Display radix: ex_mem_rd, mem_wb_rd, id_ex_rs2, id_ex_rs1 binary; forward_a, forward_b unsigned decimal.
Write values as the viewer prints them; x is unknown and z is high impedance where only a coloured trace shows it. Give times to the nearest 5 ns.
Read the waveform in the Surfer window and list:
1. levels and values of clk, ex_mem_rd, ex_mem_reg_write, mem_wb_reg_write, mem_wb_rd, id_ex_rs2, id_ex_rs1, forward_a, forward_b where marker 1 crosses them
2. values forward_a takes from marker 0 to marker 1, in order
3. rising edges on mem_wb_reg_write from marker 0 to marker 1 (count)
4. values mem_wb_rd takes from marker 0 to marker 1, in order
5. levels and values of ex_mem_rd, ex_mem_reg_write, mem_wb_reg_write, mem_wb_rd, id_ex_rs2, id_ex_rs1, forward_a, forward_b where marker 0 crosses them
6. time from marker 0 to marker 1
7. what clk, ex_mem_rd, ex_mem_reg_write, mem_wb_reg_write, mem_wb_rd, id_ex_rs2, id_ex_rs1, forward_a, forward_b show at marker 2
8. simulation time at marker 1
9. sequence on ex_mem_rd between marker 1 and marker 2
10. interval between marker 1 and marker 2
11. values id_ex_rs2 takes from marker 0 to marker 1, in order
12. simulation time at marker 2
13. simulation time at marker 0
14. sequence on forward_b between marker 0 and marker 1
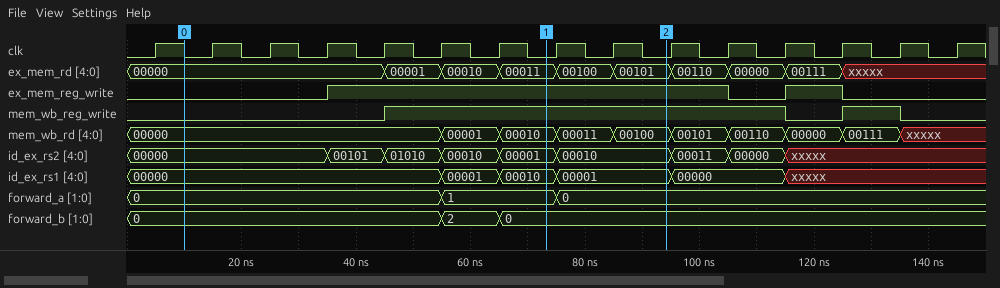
clk=0, ex_mem_rd=00011, ex_mem_reg_write=1, mem_wb_reg_write=1, mem_wb_rd=00010, id_ex_rs2=00001, id_ex_rs1=00010, forward_a=1, forward_b=0
0, 1
1
00000, 00001, 00010
ex_mem_rd=00000, ex_mem_reg_write=0, mem_wb_reg_write=0, mem_wb_rd=00000, id_ex_rs2=00000, id_ex_rs1=00000, forward_a=0, forward_b=0
65 ns
clk=0, ex_mem_rd=00101, ex_mem_reg_write=1, mem_wb_reg_write=1, mem_wb_rd=00100, id_ex_rs2=00010, id_ex_rs1=00001, forward_a=0, forward_b=0
75 ns
00011, 00100, 00101
20 ns
00000, 00101, 01010, 00010, 00001
95 ns
10 ns
0, 2, 0
